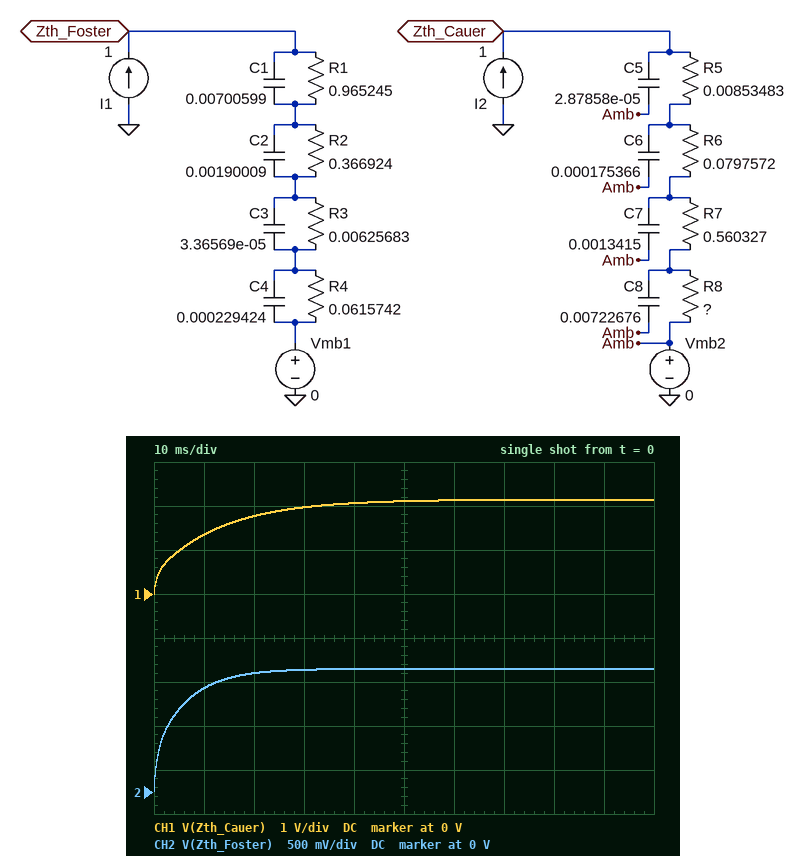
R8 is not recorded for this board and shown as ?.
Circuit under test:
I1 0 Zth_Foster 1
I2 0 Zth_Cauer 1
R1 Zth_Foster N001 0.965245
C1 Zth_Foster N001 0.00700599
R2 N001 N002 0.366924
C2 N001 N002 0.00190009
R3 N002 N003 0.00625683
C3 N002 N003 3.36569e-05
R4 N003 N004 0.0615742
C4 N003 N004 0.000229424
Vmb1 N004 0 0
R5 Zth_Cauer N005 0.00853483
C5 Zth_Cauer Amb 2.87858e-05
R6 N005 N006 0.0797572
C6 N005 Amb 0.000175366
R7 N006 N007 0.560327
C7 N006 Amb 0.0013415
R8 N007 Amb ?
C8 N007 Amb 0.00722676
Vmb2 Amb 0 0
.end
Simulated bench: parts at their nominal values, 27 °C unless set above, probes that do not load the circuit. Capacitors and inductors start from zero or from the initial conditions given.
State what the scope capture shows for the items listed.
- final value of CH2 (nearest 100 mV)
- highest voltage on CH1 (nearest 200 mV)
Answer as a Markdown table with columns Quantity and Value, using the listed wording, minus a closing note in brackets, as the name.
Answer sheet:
| Quantity | Value |
|---|---|
| final value of CH2 | 1.4 V |
| highest voltage on CH1 | 2.2 V |
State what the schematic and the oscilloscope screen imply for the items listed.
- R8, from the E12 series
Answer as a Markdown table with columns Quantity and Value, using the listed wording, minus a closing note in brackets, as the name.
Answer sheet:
| Quantity | Value |
|---|---|
| R8, from the E12 series | 1.5 Ω |
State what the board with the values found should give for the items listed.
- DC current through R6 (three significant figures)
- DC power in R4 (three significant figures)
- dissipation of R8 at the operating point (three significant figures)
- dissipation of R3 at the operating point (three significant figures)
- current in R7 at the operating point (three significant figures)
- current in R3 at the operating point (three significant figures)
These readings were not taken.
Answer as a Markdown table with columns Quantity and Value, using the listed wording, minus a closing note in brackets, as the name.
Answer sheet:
| Quantity | Value |
|---|---|
| DC current through R6 | 1.00 A |
| DC power in R4 | 61.6 mW |
| dissipation of R8 at the operating point | 1.50 W |
| dissipation of R3 at the operating point | 6.26 mW |
| current in R7 at the operating point | 1.00 A |
| current in R3 at the operating point | 1.00 A |
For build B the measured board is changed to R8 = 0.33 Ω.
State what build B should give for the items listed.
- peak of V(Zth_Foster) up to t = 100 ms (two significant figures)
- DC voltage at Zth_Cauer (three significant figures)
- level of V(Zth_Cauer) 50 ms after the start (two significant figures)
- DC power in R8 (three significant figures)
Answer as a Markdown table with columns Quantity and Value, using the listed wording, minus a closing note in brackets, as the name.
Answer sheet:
| Quantity | Value |
|---|---|
| peak of V(Zth_Foster) up to t = 100 ms | 1.4 V |
| DC voltage at Zth_Cauer | 979 mV |
| level of V(Zth_Cauer) 50 ms after the start | 980 mV |
| DC power in R8 | 330 mW |
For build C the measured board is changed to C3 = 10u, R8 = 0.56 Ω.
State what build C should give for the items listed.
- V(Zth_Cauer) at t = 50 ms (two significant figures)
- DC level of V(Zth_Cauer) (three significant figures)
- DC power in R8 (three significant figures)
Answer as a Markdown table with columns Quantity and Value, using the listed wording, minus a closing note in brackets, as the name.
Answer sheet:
| Quantity | Value |
|---|---|
| V(Zth_Cauer) at t = 50 ms | 1.2 V |
| DC level of V(Zth_Cauer) | 1.21 V |
| DC power in R8 | 560 mW |
